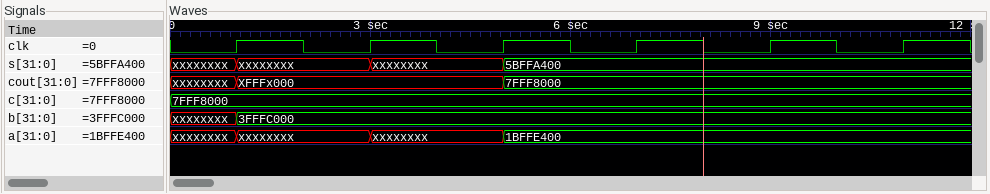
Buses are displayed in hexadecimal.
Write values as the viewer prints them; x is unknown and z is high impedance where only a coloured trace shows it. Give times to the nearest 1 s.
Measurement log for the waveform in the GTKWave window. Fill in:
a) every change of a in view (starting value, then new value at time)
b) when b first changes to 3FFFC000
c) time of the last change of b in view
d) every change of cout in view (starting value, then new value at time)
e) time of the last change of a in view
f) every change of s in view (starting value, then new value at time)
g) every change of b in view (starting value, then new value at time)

xxxxxxxx, xxxxxxxx at 1 s, xxxxxxxx at 3 s, 1BFFE400 at 5 s
1 s
1 s
xxxxxxxx, XFFFx000 at 1 s, 7FFF8000 at 5 s
5 s
xxxxxxxx, xxxxxxxx at 1 s, xxxxxxxx at 3 s, 5BFFA400 at 5 s
xxxxxxxx, 3FFFC000 at 1 s
